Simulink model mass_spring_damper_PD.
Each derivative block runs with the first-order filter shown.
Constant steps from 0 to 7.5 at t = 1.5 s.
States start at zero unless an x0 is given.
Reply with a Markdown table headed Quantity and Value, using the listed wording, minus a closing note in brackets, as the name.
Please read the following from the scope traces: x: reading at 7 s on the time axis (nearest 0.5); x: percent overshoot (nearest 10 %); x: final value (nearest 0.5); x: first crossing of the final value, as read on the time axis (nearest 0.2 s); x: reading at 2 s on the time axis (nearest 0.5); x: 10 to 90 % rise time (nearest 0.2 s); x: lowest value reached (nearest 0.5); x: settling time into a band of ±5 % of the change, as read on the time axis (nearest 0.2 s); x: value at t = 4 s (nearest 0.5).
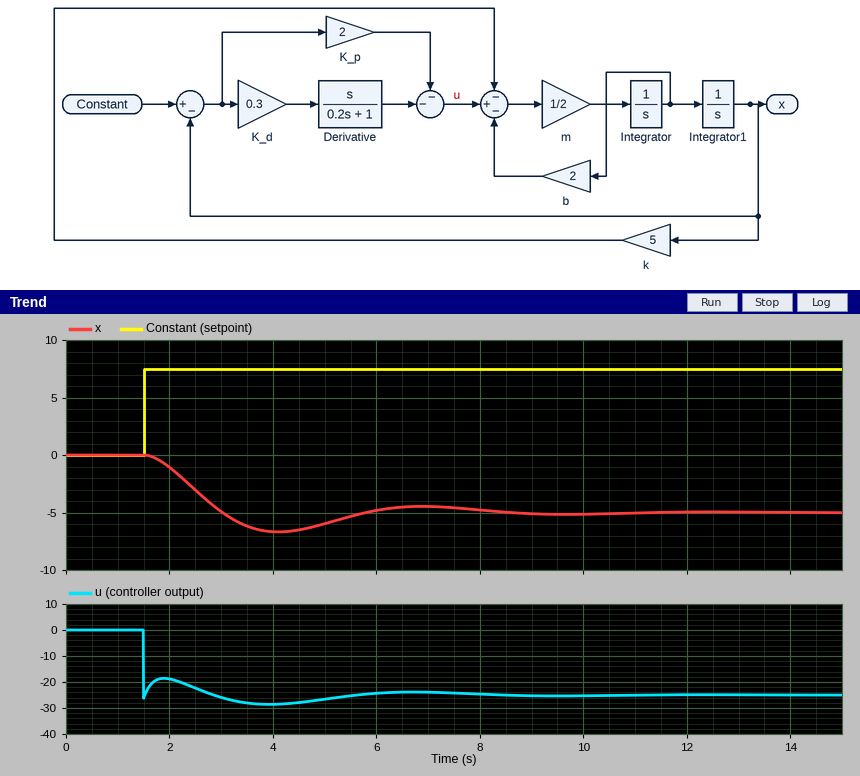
| Quantity | Value |
|---|---|
| x: reading at 7 s on the time axis | -4.5 |
| x: percent overshoot | 30 % |
| x: final value | -5.0 |
| x: first crossing of the final value, as read on the time axis | 3.0 s |
| x: reading at 2 s on the time axis | -1.0 |
| x: 10 to 90 % rise time | 1.0 s |
| x: lowest value reached | -6.5 |
| x: settling time into a band of ±5 % of the change, as read on the time axis | 8.0 s |
| x: value at t = 4 s | -6.5 |
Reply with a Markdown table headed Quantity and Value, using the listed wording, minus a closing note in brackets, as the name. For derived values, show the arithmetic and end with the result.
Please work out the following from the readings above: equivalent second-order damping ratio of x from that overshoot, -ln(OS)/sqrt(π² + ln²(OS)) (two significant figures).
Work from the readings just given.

| Quantity | Value |
|---|---|
| equivalent second-order damping ratio of x from that overshoot, -ln(OS)/sqrt(π² + ln²(OS)) | ln(0.3) = -1.204; 1.204 / sqrt(9.870 + 1.450) = 0.36 |
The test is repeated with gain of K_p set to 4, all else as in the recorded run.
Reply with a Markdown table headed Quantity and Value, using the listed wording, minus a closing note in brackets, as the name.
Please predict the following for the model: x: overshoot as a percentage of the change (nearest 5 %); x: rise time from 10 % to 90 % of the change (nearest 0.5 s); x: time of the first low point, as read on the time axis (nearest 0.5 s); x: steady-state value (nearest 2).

| Quantity | Value |
|---|---|
| x: overshoot as a percentage of the change | 10 % |
| x: rise time from 10 % to 90 % of the change | 2.5 s |
| x: time of the first low point, as read on the time axis | 7.0 s |
| x: steady-state value | -30 |
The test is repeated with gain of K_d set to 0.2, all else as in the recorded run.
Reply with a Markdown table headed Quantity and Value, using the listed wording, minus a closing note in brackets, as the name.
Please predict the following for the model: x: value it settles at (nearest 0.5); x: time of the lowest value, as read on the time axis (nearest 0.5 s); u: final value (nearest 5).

| Quantity | Value |
|---|---|
| x: value it settles at | -5.0 |
| x: time of the lowest value, as read on the time axis | 4.0 s |
| u: final value | -25 |
